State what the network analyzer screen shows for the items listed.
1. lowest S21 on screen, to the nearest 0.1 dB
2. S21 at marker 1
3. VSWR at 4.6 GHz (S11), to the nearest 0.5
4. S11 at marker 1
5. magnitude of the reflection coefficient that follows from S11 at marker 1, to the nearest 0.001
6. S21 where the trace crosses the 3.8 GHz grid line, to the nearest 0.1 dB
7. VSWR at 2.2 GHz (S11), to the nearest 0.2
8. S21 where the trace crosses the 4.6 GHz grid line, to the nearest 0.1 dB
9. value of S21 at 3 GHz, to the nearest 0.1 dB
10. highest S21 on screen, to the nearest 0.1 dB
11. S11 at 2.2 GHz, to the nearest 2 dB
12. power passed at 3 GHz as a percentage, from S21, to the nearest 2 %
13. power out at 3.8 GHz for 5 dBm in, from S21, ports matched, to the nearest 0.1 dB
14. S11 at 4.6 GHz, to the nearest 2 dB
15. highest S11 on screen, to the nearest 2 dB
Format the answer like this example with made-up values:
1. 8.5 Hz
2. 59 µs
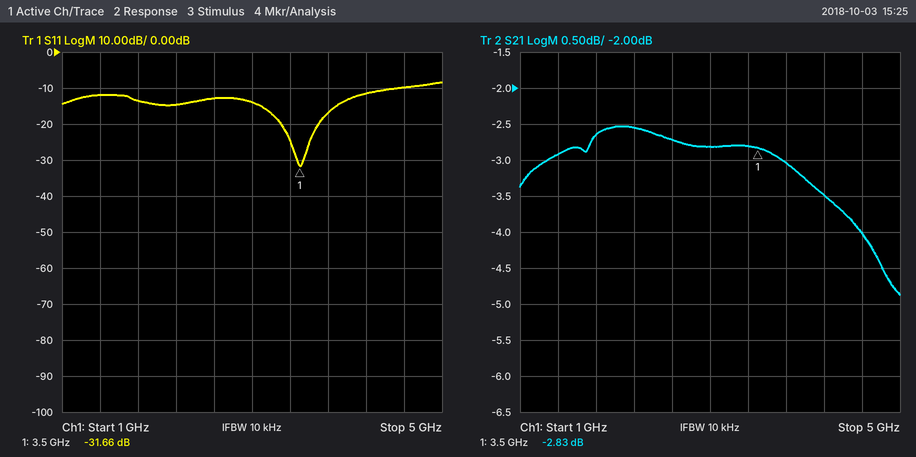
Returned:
1. -4.9 dB
2. -2.83 dB
3. 2.0
4. -31.66 dB
5. 0.026
6. -3.0 dB
7. 1.4
8. -4.0 dB
9. -2.8 dB
10. -2.5 dB
11. -14 dB
12. 52 %
13. 2.0 dBm
14. -10 dB
15. -8 dB
